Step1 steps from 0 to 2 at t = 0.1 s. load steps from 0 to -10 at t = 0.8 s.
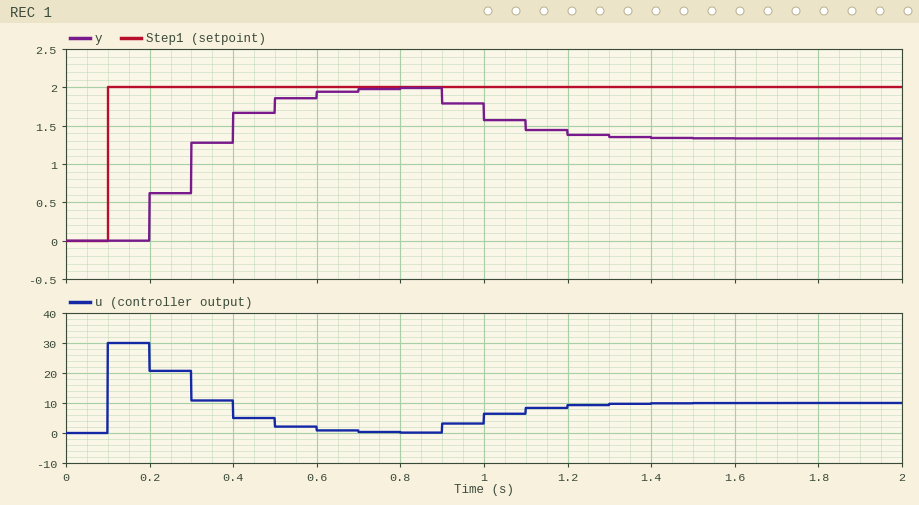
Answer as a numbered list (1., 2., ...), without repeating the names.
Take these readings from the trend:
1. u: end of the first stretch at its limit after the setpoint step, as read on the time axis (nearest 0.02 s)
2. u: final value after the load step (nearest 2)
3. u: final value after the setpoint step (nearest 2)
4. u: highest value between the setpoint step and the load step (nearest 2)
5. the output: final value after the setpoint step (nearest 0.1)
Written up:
1. 0.20 s
2. 10
3. 0
4. 30
5. 2.0
